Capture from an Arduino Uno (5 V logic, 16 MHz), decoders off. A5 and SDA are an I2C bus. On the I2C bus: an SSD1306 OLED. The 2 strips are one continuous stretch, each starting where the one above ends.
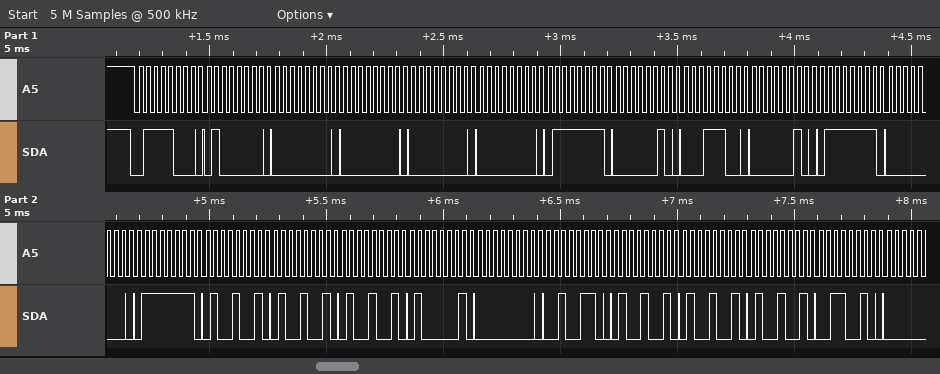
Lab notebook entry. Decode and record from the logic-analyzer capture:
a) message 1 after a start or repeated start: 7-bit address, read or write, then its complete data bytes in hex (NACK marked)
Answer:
0x3C write: 40 00 00 00 00 7F 02 1C 02 7F 00 7F 49 49 49 41 00 26 49 49 49 32
